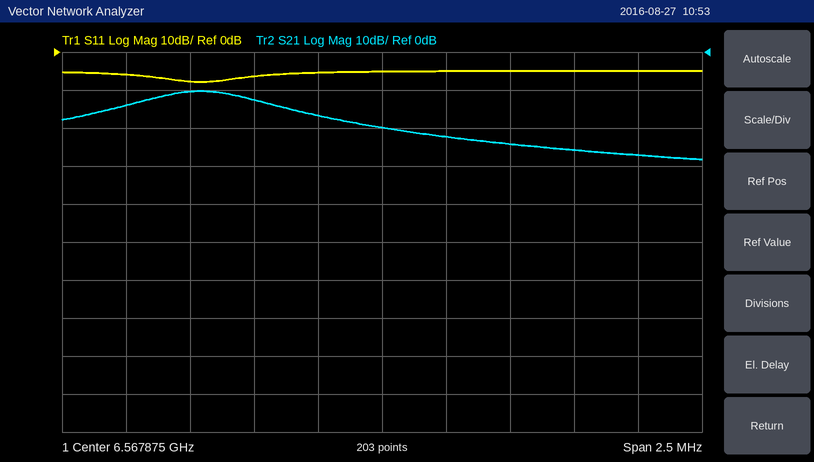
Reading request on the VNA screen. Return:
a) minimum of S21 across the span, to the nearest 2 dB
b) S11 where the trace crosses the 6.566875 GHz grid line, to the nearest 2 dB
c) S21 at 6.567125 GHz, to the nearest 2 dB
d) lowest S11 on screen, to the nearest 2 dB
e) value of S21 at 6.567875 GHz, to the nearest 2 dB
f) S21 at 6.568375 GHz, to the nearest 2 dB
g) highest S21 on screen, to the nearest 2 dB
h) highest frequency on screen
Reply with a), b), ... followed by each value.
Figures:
a) -28 dB
b) -6 dB
c) -10 dB
d) -8 dB
e) -20 dB
f) -24 dB
g) -10 dB
h) 6.569125 GHz
